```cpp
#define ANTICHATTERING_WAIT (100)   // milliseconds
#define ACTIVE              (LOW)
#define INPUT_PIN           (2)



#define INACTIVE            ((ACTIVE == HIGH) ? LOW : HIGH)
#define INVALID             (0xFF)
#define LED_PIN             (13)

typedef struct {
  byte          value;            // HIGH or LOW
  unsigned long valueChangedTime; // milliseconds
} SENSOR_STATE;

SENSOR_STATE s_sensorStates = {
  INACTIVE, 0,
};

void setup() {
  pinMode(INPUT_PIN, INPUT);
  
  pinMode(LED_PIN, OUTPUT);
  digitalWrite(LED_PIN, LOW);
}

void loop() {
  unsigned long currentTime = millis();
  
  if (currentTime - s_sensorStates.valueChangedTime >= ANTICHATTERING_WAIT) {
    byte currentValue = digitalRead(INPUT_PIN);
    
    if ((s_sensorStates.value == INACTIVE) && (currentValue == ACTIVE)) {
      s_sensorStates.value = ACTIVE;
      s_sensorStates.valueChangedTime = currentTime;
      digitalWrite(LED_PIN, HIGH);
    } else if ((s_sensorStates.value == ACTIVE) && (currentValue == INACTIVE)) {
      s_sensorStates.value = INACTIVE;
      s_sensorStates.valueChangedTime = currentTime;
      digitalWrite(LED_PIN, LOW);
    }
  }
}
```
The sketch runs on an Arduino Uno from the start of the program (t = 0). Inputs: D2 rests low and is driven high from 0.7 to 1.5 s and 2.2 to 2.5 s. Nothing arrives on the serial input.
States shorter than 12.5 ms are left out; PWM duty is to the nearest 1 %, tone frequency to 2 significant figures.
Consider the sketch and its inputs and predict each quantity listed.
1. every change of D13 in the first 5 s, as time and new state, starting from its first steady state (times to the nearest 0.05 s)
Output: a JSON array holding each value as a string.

["0 s low; 0.1 s high; 0.7 s low; 1.5 s high; 2.2 s low; 2.5 s high"]
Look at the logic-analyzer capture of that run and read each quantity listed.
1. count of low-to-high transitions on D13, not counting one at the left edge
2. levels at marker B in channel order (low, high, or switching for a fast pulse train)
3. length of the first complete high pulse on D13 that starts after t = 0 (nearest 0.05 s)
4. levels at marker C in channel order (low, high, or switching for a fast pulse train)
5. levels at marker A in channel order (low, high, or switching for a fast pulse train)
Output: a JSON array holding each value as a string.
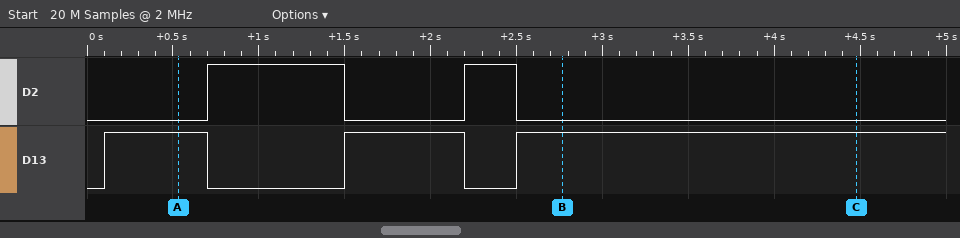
["3", "D2 low, D13 high", "0.60 s", "D2 low, D13 high", "D2 low, D13 high"]
